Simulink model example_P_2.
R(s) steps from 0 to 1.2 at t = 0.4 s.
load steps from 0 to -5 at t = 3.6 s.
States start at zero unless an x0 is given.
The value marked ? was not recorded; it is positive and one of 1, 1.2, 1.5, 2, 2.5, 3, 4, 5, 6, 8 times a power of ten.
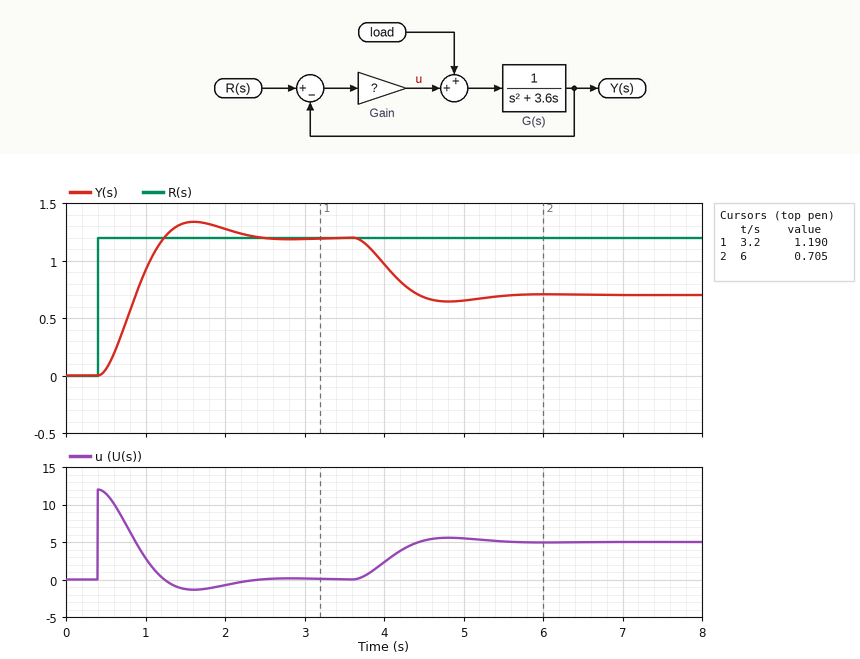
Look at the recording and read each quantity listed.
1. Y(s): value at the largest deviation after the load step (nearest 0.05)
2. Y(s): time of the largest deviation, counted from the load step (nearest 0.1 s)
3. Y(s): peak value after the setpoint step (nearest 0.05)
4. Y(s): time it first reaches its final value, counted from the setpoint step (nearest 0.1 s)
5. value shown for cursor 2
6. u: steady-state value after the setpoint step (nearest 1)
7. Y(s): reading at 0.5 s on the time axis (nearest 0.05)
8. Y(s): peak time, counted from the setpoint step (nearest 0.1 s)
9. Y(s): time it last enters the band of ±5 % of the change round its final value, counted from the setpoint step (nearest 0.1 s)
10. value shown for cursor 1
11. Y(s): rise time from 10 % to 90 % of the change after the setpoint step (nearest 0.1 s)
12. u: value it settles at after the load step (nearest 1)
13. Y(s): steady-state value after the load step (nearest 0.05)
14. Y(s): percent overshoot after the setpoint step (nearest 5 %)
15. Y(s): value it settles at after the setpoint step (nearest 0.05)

0.65
1.2 s
1.35
0.8 s
0.705
0
0.05
1.2 s
1.7 s
1.190
0.6 s
5
0.70
10 %
1.20
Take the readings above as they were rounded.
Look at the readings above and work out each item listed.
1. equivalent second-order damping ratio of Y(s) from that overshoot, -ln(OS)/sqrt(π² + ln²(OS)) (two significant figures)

0.59
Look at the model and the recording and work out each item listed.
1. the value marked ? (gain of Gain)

10
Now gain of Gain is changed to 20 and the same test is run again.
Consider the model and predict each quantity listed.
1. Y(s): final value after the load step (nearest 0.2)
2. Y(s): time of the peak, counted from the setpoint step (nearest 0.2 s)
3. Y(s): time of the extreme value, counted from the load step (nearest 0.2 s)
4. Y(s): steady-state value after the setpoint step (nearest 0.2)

1.0
0.8 s
0.8 s
1.2
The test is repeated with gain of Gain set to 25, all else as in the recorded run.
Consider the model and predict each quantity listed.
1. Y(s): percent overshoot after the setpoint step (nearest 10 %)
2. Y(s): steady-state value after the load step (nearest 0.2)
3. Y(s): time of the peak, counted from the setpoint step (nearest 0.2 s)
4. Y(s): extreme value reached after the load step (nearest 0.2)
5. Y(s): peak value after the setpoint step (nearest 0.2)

30 %
1.0
0.6 s
1.0
1.6
